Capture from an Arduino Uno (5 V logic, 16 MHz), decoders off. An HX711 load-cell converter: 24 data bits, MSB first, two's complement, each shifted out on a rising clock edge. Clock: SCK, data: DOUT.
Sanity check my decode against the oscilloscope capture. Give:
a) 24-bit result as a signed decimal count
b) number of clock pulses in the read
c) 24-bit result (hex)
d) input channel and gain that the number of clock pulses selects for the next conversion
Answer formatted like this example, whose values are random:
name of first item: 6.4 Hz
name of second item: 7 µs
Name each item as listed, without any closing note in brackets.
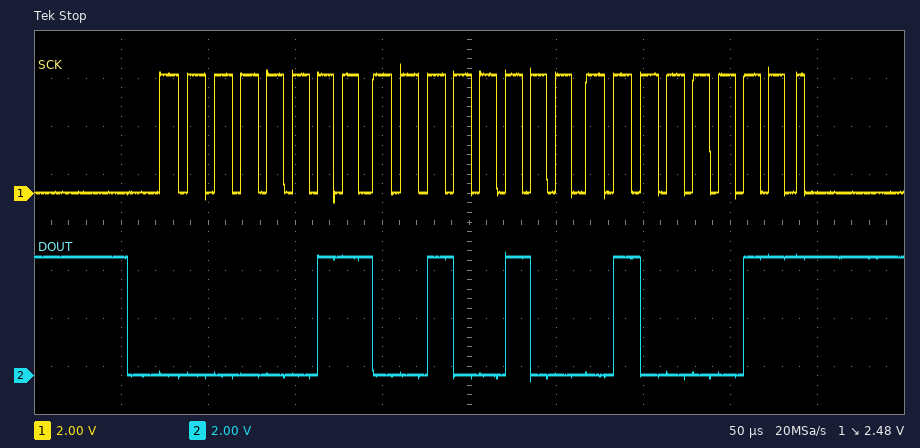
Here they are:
24-bit result as a signed decimal count: 205891
number of clock pulses in the read: 25
24-bit result: 0x032443
input channel and gain that the number of clock pulses selects for the next conversion: channel A, gain 128
